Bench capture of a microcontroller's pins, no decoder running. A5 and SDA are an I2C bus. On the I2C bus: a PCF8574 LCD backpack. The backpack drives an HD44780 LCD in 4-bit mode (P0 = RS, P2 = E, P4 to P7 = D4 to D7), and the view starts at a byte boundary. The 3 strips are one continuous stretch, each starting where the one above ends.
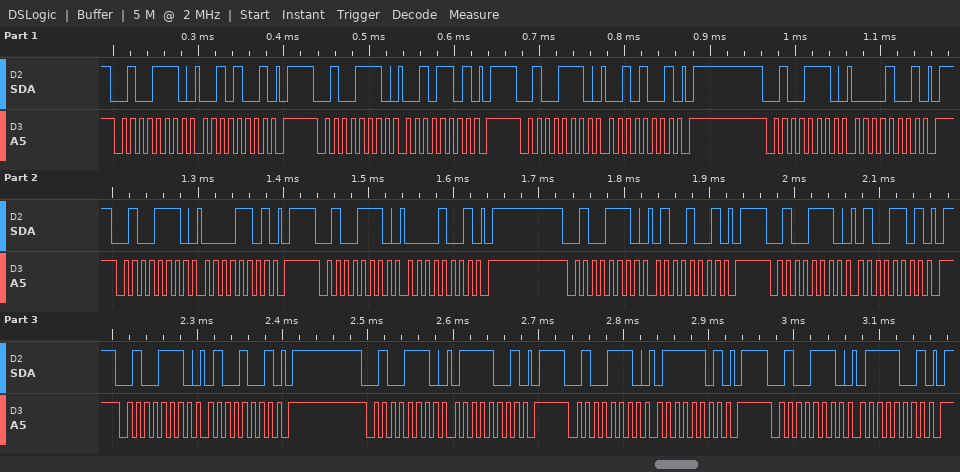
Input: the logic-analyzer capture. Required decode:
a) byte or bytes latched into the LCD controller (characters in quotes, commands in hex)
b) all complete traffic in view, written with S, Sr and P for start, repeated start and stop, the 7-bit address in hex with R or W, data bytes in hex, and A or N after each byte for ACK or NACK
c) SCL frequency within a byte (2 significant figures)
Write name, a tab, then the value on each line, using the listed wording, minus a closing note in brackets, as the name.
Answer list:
byte or bytes latched into the LCD controller	' ' 'G'
all complete traffic in view, written with S, Sr and P for start, repeated start and stop, the 7-bit address in hex with R or W, data bytes in hex, and A or N after each byte for ACK or NACK	S 27W A 29 A P S 27W A 2D A P S 27W A 29 A P S 27W A 09 A P S 27W A 0D A P S 27W A 09 A P S 27W A 49 A P S 27W A 4D A P S 27W A 49 A P S 27W A 79 A P S 27W A 7D A P S 27W A 79 A P
SCL frequency within a byte	100 kHz
